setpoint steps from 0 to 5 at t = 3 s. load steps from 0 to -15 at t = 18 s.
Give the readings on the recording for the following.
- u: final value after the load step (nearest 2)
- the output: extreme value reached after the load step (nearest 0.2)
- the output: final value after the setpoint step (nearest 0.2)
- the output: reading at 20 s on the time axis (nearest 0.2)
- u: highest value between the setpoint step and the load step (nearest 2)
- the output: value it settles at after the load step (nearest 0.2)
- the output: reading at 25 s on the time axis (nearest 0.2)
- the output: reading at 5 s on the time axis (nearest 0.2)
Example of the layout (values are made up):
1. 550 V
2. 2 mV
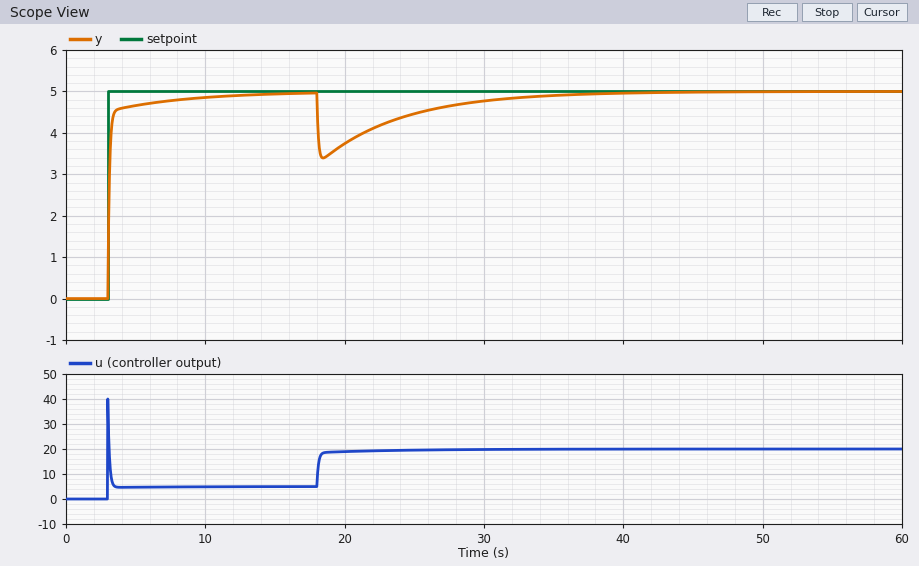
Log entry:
1. 20
2. 3.4
3. 5.0
4. 3.8
5. 40
6. 5.0
7. 4.4
8. 4.6
